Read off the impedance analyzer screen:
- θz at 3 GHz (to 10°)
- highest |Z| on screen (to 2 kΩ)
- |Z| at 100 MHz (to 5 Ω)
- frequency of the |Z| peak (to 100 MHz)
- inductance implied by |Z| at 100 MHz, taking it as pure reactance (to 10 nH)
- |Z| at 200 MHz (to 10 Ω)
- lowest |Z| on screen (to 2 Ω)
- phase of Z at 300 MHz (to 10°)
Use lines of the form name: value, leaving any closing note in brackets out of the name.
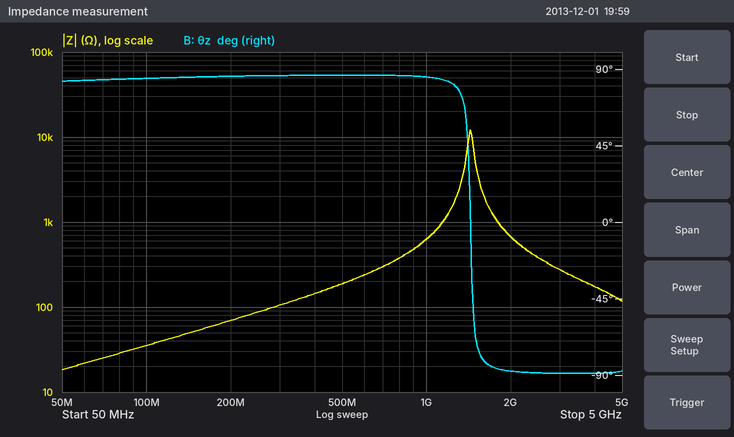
θz at 3 GHz: -90°
highest |Z| on screen: 12 kΩ
|Z| at 100 MHz: 35 Ω
frequency of the |Z| peak: 1.4 GHz
inductance implied by |Z| at 100 MHz, taking it as pure reactance: 60 nH
|Z| at 200 MHz: 70 Ω
lowest |Z| on screen: 18 Ω
phase of Z at 300 MHz: 90°
